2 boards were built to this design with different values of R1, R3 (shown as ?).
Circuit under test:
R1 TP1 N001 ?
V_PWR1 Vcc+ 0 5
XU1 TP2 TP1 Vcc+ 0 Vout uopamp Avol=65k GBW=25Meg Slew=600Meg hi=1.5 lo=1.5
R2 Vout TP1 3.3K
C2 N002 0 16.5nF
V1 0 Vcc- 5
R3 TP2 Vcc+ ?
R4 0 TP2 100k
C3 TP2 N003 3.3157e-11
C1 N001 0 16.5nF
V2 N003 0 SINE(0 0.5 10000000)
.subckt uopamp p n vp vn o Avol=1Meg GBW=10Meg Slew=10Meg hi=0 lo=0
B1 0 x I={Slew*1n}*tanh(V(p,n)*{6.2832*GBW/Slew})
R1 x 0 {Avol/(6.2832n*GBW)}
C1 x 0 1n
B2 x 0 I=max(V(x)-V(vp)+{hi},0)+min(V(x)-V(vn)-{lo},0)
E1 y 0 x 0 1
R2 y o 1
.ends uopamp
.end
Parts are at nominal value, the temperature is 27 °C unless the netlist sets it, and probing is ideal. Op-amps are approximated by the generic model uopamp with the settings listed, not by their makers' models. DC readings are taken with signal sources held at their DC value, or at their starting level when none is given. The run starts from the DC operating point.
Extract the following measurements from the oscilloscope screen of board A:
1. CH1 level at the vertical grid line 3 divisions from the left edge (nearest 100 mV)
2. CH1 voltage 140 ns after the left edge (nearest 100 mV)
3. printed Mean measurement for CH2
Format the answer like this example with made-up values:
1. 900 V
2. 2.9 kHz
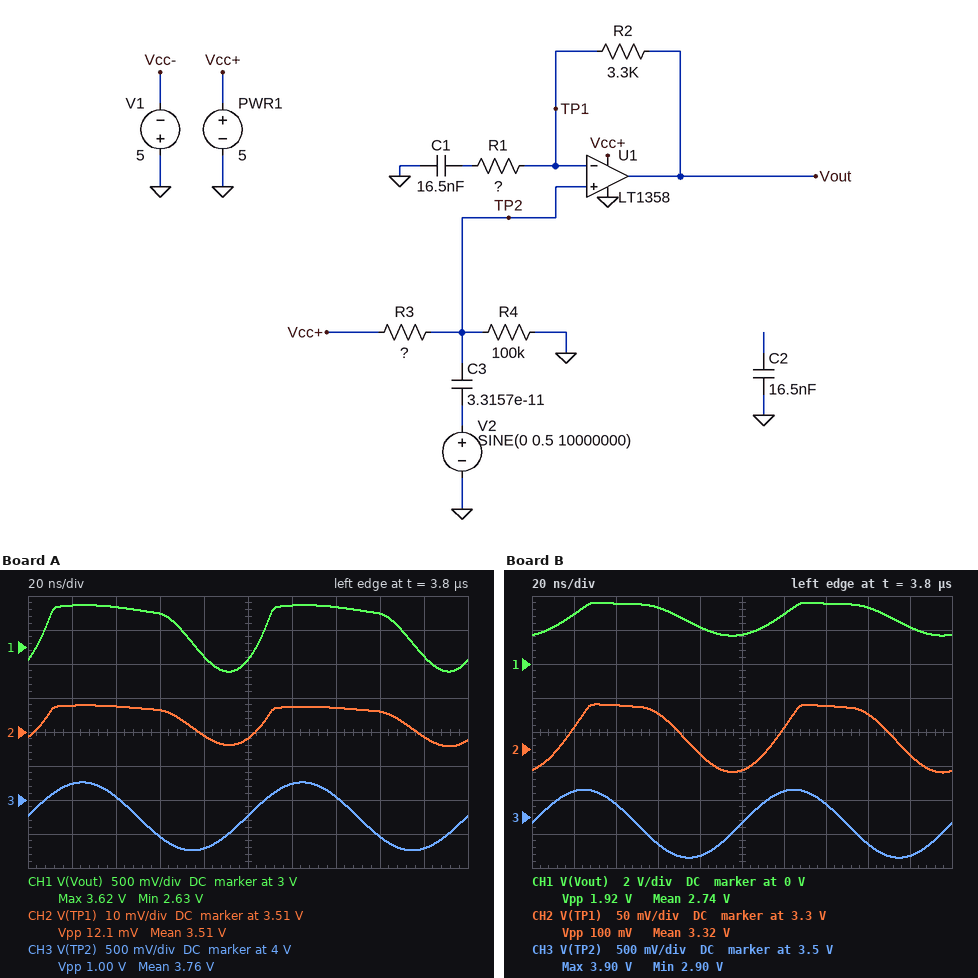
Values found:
1. 3.5 V
2. 3.6 V
3. 3.51 V
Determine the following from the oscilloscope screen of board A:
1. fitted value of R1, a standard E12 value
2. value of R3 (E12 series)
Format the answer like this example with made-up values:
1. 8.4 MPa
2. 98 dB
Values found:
1. 39 Ω
2. 33 kΩ
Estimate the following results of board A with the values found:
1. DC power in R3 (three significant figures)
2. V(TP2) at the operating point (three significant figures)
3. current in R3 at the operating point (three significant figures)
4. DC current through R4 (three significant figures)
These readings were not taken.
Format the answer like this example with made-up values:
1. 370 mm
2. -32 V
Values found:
1. 46.6 µW
2. 3.76 V
3. 37.6 µA
4. 37.6 µA
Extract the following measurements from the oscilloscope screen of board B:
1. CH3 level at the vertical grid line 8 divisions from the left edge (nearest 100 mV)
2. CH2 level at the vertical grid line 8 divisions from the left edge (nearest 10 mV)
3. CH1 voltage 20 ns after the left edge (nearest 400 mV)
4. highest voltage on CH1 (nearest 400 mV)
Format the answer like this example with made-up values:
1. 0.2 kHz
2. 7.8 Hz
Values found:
1. 3.1 V
2. 3.35 V
3. 2.8 V
4. 3.6 V
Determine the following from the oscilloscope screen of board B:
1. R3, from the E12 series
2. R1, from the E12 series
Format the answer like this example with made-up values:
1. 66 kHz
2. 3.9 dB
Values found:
1. 47 kΩ
2. 180 Ω
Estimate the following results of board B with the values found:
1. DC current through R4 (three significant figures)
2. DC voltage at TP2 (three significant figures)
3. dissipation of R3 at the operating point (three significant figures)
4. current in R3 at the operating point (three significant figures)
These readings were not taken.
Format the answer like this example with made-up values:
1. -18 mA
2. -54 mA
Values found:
1. 34.0 µA
2. 3.40 V
3. 54.4 µW
4. 34.0 µA
